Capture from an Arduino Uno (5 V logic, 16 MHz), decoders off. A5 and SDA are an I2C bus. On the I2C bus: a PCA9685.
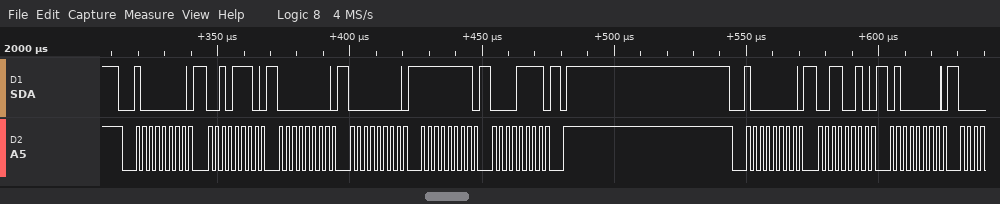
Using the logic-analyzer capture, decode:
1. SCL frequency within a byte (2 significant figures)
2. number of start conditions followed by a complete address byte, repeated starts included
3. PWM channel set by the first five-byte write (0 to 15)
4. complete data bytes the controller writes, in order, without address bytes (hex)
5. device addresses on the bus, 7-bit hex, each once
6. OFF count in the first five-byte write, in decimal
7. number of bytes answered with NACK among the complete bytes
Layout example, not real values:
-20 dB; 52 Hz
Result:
400 kHz; 2; 10; 2E 00 00 FF 0F 32 40; 0x40; 4095; 0
